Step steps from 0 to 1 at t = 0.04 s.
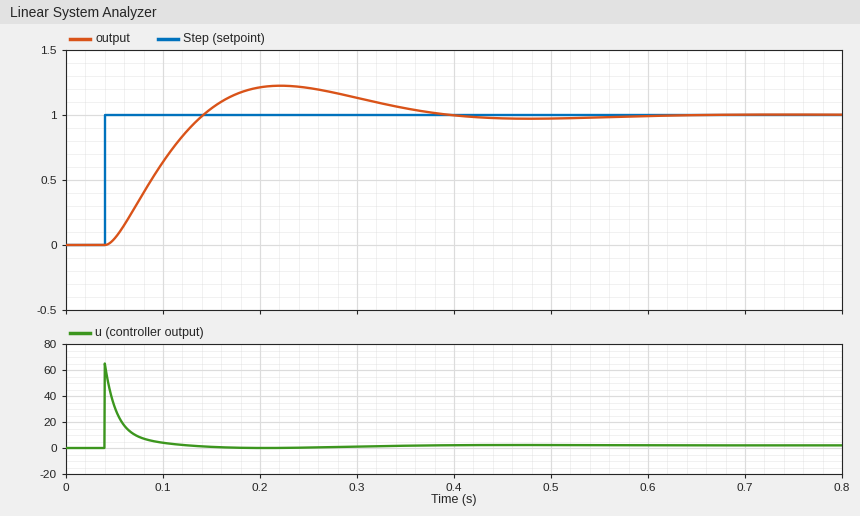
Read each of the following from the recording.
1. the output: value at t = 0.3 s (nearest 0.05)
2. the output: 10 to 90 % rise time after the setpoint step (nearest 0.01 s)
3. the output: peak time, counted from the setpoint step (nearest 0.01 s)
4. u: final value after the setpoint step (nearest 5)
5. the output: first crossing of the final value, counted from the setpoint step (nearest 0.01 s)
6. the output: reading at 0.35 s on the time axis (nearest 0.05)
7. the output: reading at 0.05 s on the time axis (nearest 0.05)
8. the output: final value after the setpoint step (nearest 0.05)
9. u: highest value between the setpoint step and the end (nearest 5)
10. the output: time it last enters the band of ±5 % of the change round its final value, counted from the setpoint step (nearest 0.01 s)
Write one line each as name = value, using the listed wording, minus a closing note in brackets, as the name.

the output: value at t = 0.3 s = 1.15
the output: 10 to 90 % rise time after the setpoint step = 0.07 s
the output: peak time, counted from the setpoint step = 0.18 s
u: final value after the setpoint step = 0
the output: first crossing of the final value, counted from the setpoint step = 0.10 s
the output: reading at 0.35 s on the time axis = 1.05
the output: reading at 0.05 s on the time axis = 0.05
the output: final value after the setpoint step = 1.00
u: highest value between the setpoint step and the end = 65
the output: time it last enters the band of ±5 % of the change round its final value, counted from the setpoint step = 0.31 s
